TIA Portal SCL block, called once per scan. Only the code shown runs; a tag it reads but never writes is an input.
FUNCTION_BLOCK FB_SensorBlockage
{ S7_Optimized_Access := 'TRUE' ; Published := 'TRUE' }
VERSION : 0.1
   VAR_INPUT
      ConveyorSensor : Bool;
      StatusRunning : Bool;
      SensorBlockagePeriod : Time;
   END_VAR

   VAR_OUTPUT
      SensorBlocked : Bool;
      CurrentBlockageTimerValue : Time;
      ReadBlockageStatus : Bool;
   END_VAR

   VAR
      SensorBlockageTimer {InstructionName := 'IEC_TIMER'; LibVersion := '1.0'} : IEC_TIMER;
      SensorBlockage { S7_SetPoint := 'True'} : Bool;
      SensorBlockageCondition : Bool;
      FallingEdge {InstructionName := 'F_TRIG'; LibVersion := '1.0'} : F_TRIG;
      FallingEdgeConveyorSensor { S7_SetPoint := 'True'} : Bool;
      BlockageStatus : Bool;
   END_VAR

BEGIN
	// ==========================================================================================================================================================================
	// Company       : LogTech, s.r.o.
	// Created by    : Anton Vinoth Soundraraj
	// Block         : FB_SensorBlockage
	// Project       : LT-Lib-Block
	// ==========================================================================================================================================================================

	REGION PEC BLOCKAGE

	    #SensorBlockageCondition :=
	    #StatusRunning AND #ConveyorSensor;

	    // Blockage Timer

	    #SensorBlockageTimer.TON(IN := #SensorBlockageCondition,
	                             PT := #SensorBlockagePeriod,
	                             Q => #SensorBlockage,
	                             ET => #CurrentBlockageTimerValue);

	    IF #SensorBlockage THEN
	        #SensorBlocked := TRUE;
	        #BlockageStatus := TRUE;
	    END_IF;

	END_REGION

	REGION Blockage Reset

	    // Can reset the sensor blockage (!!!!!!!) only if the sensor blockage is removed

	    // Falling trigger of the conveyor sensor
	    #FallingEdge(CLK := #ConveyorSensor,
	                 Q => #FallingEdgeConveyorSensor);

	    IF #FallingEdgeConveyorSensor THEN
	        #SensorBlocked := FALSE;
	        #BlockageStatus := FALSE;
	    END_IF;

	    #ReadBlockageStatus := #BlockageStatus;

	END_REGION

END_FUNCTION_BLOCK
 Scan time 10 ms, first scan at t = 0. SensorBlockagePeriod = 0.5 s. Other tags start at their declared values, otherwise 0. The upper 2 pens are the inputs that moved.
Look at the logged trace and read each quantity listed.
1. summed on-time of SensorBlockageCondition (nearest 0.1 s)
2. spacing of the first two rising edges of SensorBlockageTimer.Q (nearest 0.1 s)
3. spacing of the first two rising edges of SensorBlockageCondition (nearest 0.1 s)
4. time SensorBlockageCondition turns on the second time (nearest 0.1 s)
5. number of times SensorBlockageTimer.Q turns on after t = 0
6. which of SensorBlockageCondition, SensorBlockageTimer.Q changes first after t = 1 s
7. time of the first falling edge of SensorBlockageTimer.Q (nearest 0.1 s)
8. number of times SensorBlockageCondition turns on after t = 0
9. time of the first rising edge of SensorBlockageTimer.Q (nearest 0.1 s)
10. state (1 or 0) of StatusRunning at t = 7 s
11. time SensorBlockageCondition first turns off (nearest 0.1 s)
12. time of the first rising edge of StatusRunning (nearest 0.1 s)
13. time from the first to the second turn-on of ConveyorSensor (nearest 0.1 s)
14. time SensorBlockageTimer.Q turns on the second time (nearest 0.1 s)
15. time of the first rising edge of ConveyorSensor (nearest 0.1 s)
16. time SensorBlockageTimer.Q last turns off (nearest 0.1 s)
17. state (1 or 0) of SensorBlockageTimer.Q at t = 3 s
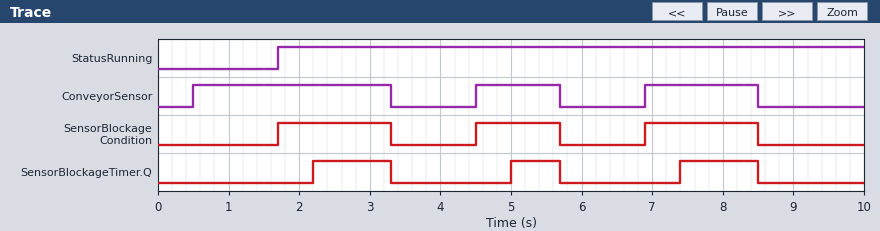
4.4 s
2.8 s
2.8 s
4.5 s
3
SensorBlockageCondition
3.3 s
3
2.2 s
1
3.3 s
1.7 s
4.0 s
5.0 s
0.5 s
8.5 s
1
